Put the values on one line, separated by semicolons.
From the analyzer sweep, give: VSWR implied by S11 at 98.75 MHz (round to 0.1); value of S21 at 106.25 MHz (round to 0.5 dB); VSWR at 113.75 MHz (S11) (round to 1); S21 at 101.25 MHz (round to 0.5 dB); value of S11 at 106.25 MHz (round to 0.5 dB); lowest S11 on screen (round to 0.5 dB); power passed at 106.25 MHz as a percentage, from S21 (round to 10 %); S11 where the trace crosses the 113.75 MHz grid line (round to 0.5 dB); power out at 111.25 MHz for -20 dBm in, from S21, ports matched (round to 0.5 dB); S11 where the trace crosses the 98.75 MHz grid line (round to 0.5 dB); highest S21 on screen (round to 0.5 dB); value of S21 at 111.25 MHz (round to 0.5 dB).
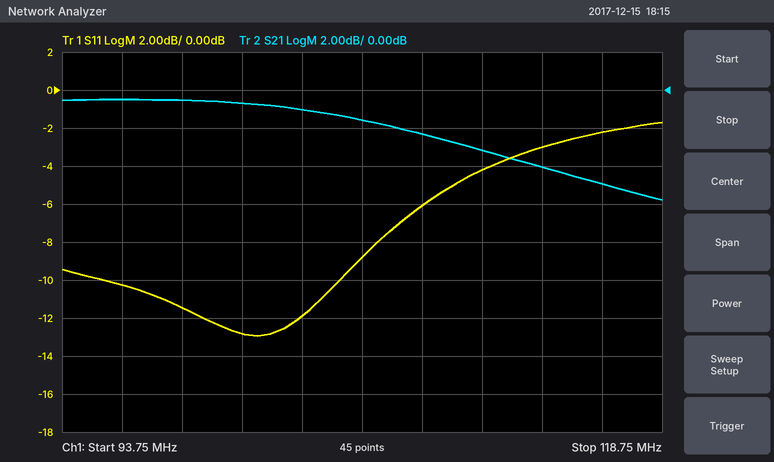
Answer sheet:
1.7; -1.5 dB; 6; -0.5 dB; -9.0 dB; -13.0 dB; 70 %; -3.0 dB; -23.0 dBm; -11.5 dB; -0.5 dB; -3.0 dB
